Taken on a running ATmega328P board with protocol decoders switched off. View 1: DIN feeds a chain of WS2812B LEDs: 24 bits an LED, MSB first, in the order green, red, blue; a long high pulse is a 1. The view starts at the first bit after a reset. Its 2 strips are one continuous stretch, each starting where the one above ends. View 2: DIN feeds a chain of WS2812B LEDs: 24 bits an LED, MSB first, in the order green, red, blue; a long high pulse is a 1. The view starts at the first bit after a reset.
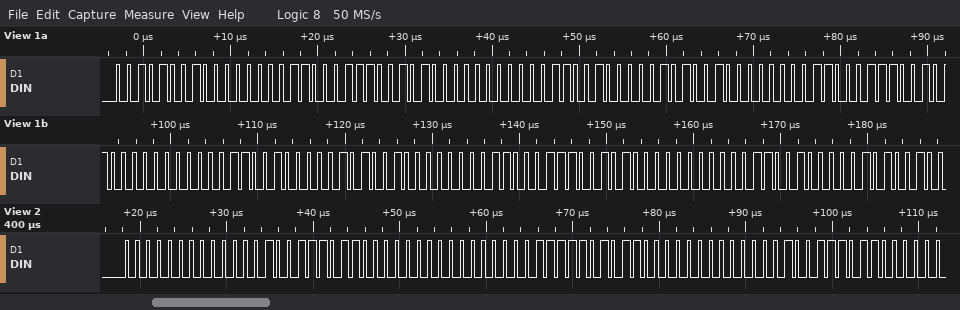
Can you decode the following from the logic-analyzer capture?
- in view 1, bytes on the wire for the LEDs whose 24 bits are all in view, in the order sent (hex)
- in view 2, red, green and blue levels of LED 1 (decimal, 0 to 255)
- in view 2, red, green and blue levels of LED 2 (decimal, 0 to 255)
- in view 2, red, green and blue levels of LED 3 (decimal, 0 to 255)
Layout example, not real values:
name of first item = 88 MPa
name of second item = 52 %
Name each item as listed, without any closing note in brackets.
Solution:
in view 1, bytes on the wire for the LEDs whose 24 bits are all in view, in the order sent = 29 00 C7 28 00 C8 29 00 C7 28 00 C8 29 00 C7 28 00 C8
in view 2, red, green and blue levels of LED 1 = 4, 0, 236
in view 2, red, green and blue levels of LED 2 = 3, 0, 235
in view 2, red, green and blue levels of LED 3 = 4, 0, 236
